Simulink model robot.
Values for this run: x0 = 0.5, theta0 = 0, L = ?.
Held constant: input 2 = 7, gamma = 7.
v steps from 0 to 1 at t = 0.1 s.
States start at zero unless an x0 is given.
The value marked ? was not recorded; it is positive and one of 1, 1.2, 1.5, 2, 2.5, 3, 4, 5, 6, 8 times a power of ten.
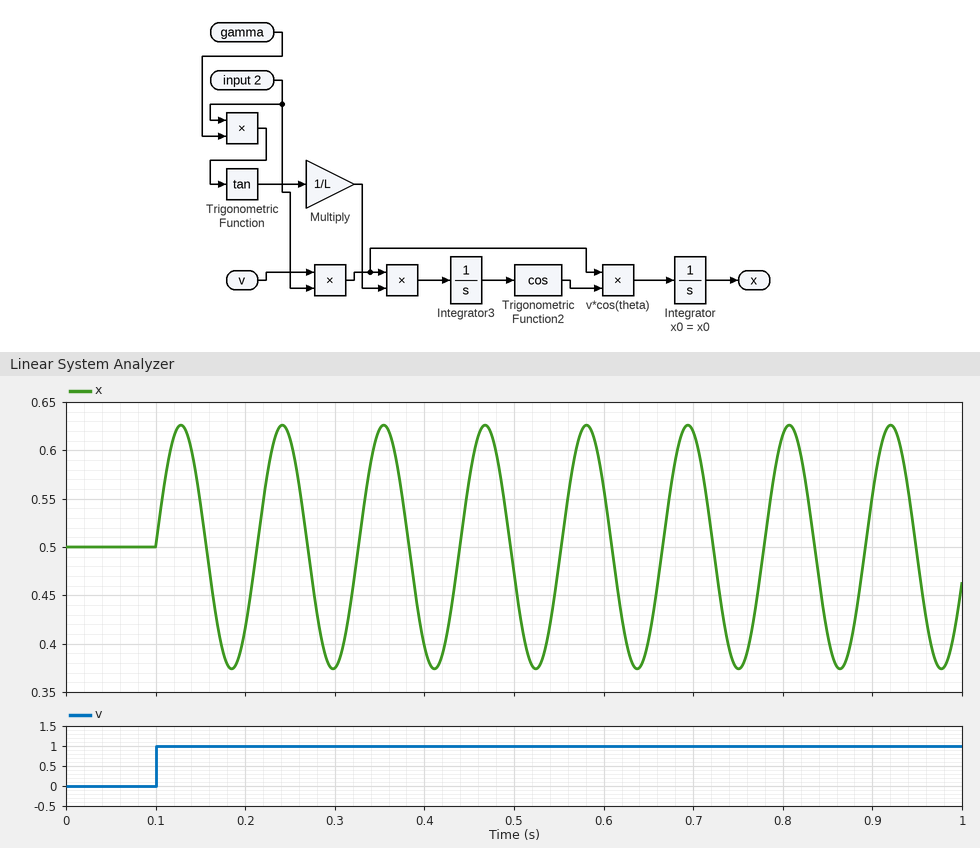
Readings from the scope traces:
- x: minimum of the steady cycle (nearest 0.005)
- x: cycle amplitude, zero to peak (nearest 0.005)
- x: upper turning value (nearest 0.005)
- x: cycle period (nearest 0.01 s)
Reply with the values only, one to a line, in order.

0.375
0.125
0.625
0.11 s
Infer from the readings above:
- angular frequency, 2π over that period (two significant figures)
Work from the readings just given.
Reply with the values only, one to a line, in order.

57 rad/s
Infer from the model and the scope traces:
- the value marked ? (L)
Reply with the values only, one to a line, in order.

0.4
